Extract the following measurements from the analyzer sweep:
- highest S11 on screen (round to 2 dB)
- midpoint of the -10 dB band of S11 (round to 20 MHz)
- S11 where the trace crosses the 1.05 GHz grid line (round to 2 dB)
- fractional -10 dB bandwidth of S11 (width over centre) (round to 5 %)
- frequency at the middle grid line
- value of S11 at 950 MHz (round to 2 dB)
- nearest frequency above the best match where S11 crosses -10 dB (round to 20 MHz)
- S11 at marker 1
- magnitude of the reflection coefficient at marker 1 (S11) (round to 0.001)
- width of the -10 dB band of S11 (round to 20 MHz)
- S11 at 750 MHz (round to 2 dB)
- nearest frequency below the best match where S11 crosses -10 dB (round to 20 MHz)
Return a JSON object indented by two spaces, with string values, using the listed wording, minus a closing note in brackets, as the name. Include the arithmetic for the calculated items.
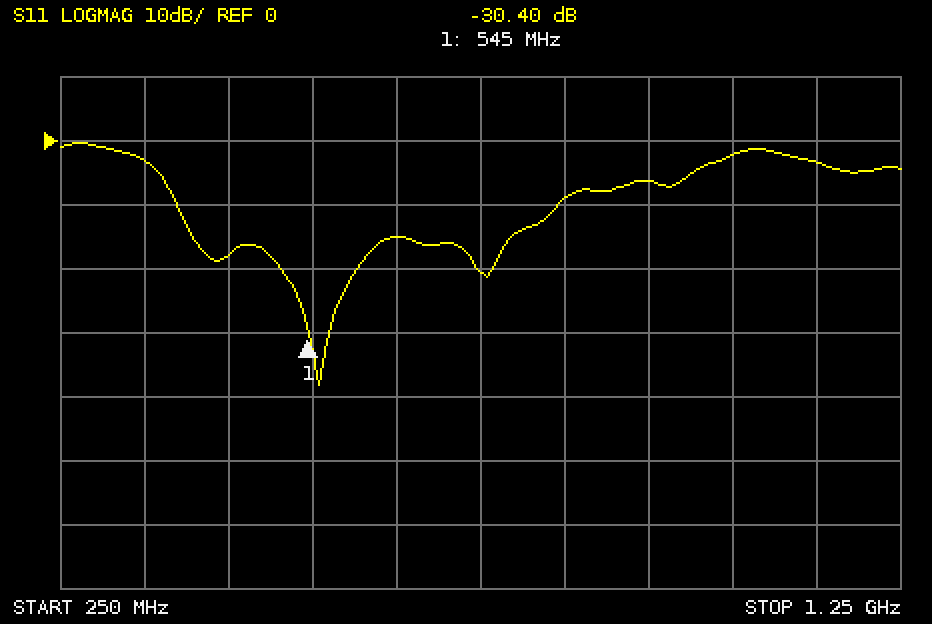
{
  "highest S11 on screen": "0 dB",
  "midpoint of the -10 dB band of S11": "620 MHz",
  "S11 where the trace crosses the 1.05 GHz grid line": "-2 dB",
  "fractional -10 dB bandwidth of S11 (width over centre)": "460 MHz / 610 MHz ≈ 75 %",
  "frequency at the middle grid line": "750 MHz",
  "value of S11 at 950 MHz": "-6 dB",
  "nearest frequency above the best match where S11 crosses -10 dB": "840 MHz",
  "S11 at marker 1": "-30.40 dB",
  "magnitude of the reflection coefficient at marker 1 (S11)": "10^(-30.4/20) ≈ 0.030",
  "width of the -10 dB band of S11": "840 MHz − 380 MHz = 460 MHz",
  "S11 at 750 MHz": "-20 dB",
  "nearest frequency below the best match where S11 crosses -10 dB": "380 MHz"
}
